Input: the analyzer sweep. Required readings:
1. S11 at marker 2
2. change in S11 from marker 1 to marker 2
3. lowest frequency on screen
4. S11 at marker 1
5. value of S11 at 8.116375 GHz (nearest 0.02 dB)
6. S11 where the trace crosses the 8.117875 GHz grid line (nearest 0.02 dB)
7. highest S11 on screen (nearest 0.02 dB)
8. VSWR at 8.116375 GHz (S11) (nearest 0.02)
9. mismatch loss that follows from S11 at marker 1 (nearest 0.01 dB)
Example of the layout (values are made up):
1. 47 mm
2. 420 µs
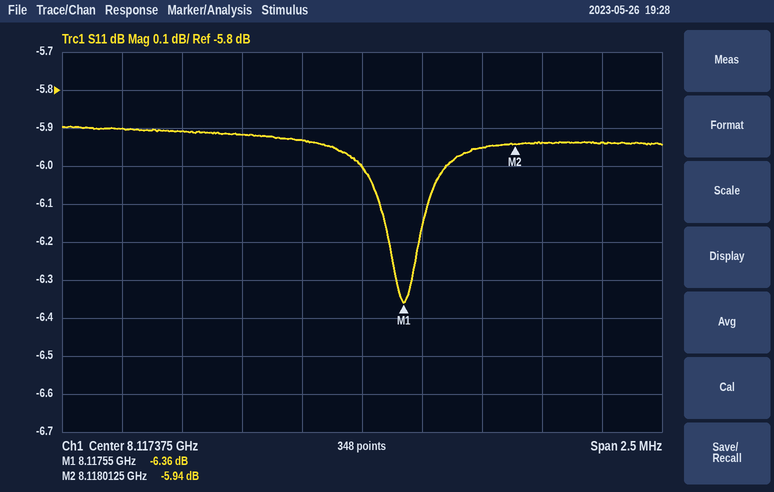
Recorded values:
1. -5.94 dB
2. 0.42 dB
3. 8.116125 GHz
4. -6.36 dB
5. -5.90 dB
6. -5.96 dB
7. -5.90 dB
8. 3.06
9. 1.14 dB
